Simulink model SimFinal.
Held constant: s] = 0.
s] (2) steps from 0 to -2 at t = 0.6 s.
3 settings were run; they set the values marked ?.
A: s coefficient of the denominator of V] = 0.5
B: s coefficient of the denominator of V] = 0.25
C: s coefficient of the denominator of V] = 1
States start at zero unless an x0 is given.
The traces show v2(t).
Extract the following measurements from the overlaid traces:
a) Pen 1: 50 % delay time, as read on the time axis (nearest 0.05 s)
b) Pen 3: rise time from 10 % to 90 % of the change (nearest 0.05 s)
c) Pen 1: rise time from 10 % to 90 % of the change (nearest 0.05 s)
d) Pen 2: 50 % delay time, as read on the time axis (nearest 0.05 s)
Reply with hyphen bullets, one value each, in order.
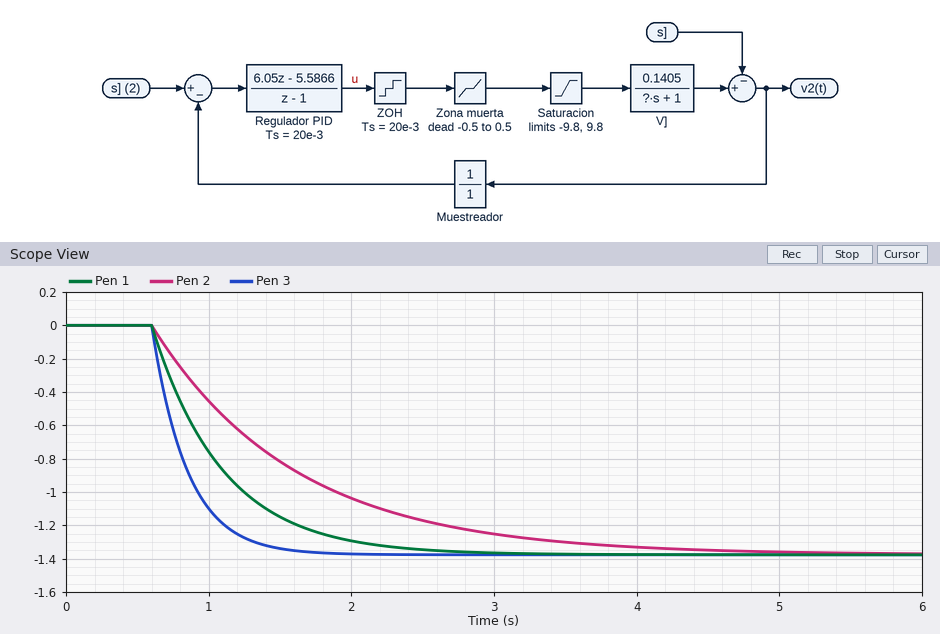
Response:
- 0.95 s
- 0.55 s
- 1.10 s
- 1.30 s
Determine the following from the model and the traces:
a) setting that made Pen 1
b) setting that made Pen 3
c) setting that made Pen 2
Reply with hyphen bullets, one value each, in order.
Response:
- A
- B
- C
